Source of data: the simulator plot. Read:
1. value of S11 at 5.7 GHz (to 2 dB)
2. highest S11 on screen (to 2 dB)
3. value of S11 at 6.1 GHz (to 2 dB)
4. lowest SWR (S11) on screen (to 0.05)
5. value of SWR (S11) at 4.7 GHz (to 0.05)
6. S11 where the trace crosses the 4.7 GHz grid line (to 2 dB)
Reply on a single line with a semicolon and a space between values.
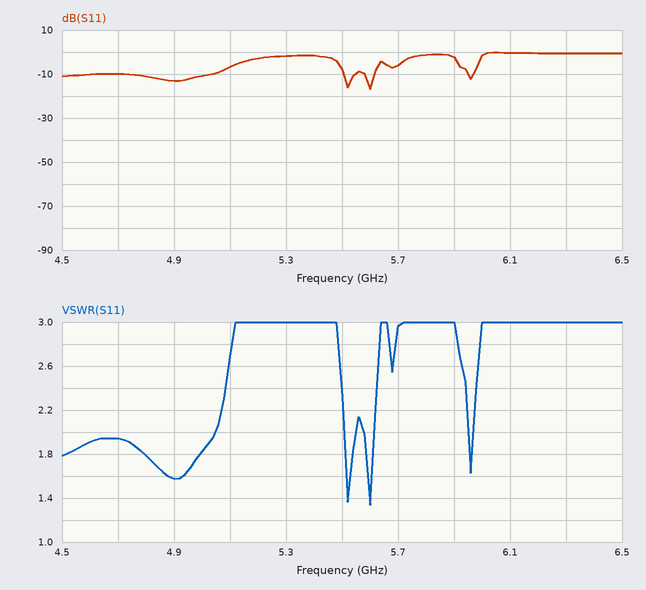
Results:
-6 dB; 0 dB; 0 dB; 1.35; 1.95; -10 dB
